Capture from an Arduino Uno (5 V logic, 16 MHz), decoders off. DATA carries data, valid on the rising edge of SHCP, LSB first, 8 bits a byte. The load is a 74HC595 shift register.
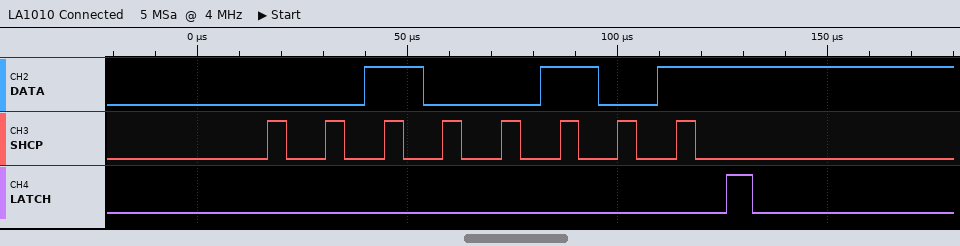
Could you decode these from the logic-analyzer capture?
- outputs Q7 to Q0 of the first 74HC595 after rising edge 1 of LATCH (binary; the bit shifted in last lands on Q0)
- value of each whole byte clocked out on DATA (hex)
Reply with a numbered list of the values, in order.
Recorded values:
1. 00100101
2. A4
